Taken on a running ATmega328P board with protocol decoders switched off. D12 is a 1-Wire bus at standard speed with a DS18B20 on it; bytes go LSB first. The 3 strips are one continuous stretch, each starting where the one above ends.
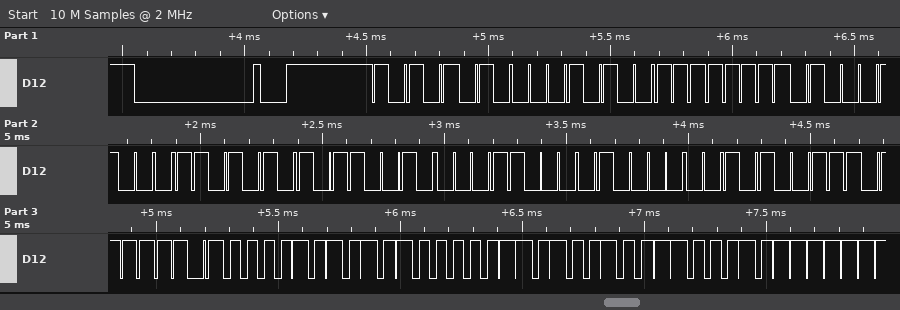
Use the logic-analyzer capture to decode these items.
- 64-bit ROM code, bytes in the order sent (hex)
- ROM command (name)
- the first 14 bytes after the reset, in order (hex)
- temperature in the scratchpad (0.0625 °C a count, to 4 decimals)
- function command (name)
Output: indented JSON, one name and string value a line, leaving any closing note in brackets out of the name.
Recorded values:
{
  "64-bit ROM code, bytes in the order sent": "28 FF 22 56 4D 18 02 E5",
  "ROM command": "Match ROM",
  "the first 14 bytes after the reset, in order": "55 28 FF 22 56 4D 18 02 E5 BE 50 05 4B 46",
  "temperature in the scratchpad": "85.0000 °C",
  "function command": "Read Scratchpad"
}
